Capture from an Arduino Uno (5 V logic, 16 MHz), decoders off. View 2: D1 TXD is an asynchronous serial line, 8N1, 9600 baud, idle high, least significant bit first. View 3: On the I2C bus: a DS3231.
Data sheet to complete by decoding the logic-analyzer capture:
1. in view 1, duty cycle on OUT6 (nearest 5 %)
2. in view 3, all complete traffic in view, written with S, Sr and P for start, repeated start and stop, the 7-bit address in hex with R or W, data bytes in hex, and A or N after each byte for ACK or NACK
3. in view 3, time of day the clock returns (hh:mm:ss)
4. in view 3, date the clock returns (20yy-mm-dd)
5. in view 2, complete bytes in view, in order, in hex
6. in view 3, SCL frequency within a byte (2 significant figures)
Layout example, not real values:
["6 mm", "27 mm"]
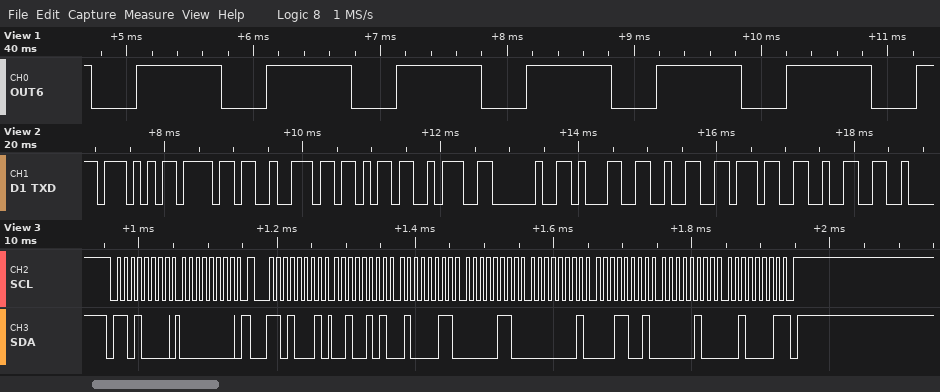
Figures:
["65 %", "S 68W A 00 A Sr 68R A 25 A 43 A 06 A 01 A 19 A 04 A 21 N P", "06:43:25", "2021-04-19", "57 6F 72 6B 3A 20 31 32 37 32", "100 kHz"]
